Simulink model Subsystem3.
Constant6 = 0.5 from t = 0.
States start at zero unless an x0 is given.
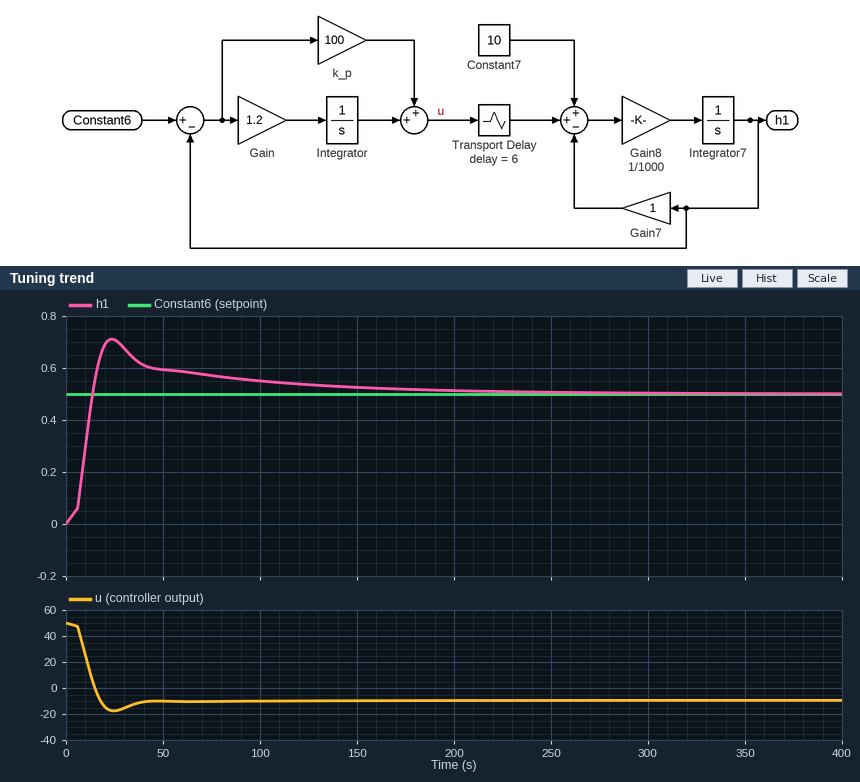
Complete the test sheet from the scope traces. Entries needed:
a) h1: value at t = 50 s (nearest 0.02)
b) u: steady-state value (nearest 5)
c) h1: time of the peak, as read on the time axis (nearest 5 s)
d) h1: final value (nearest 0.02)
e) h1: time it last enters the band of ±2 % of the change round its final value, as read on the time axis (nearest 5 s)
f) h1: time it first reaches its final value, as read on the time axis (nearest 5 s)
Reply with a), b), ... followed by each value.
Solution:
a) 0.60
b) -10
c) 25 s
d) 0.50
e) 220 s
f) 15 s
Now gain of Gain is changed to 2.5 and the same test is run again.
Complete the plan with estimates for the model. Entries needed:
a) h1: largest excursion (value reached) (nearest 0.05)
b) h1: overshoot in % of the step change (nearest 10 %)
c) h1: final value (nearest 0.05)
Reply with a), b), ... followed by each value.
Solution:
a) 0.75
b) 50 %
c) 0.50
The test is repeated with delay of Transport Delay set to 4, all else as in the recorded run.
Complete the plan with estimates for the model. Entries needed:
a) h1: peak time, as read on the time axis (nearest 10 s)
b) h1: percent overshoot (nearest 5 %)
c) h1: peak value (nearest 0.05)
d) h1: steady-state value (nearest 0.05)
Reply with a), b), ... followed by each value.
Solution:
a) 30 s
b) 25 %
c) 0.65
d) 0.50
